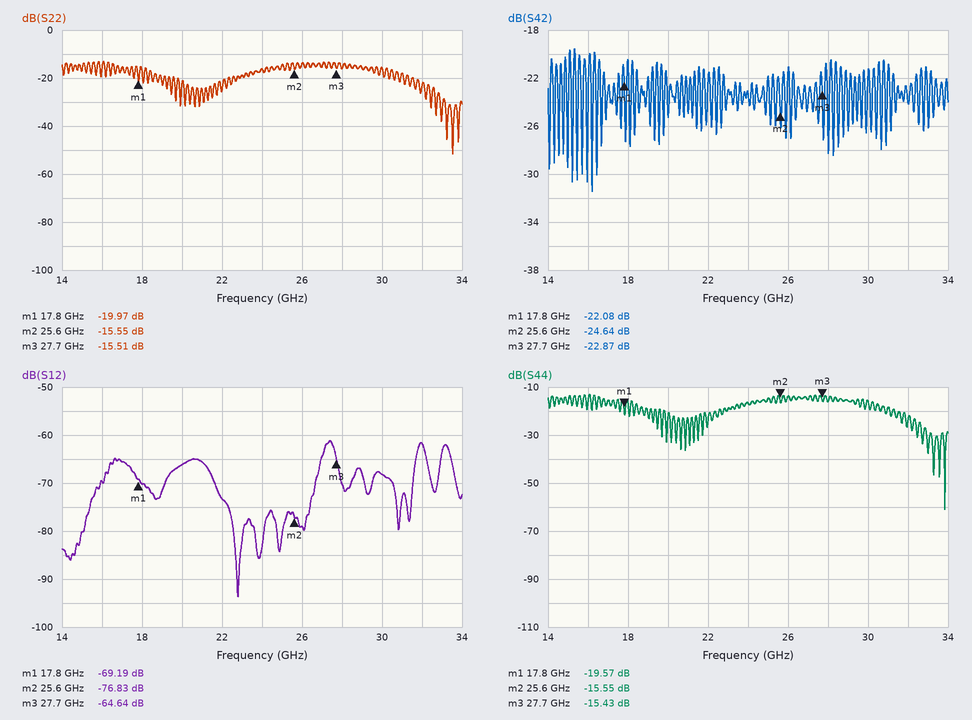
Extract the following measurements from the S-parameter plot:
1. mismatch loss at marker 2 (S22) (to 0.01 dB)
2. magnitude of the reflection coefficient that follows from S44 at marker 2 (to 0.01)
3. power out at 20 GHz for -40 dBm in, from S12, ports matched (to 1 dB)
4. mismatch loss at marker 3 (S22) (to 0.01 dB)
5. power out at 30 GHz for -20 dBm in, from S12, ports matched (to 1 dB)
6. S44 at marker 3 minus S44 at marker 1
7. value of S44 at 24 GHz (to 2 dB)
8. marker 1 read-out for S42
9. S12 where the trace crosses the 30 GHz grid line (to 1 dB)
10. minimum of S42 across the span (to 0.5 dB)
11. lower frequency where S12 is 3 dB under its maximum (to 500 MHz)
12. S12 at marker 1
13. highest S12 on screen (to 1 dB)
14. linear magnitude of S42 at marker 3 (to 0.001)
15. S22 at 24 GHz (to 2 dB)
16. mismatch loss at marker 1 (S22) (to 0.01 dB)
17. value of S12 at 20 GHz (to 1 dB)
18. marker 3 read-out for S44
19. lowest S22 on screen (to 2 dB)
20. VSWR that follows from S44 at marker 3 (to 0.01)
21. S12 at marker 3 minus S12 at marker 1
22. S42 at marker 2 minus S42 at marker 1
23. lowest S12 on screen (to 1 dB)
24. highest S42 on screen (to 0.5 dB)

0.12 dB
0.17
-106 dBm
0.12 dB
-88 dBm
4.14 dB
-16 dB
-22.08 dB
-68 dB
-31.5 dB
27.0 GHz
-69.19 dB
-61 dB
0.072
-16 dB
0.04 dB
-66 dB
-15.43 dB
-52 dB
1.41
4.55 dB
-2.56 dB
-94 dB
-19.5 dB
